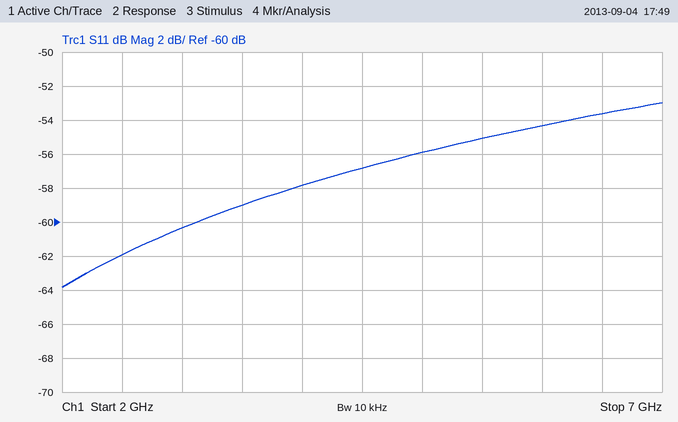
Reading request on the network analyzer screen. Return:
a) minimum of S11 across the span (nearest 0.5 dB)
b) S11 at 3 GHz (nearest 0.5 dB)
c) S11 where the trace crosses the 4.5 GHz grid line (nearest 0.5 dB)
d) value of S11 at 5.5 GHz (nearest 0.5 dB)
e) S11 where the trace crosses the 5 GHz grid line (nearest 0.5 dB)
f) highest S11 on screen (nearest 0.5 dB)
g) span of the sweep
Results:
-64.0 dB
-60.5 dB
-57.0 dB
-55.0 dB
-56.0 dB
-53.0 dB
5 GHz
